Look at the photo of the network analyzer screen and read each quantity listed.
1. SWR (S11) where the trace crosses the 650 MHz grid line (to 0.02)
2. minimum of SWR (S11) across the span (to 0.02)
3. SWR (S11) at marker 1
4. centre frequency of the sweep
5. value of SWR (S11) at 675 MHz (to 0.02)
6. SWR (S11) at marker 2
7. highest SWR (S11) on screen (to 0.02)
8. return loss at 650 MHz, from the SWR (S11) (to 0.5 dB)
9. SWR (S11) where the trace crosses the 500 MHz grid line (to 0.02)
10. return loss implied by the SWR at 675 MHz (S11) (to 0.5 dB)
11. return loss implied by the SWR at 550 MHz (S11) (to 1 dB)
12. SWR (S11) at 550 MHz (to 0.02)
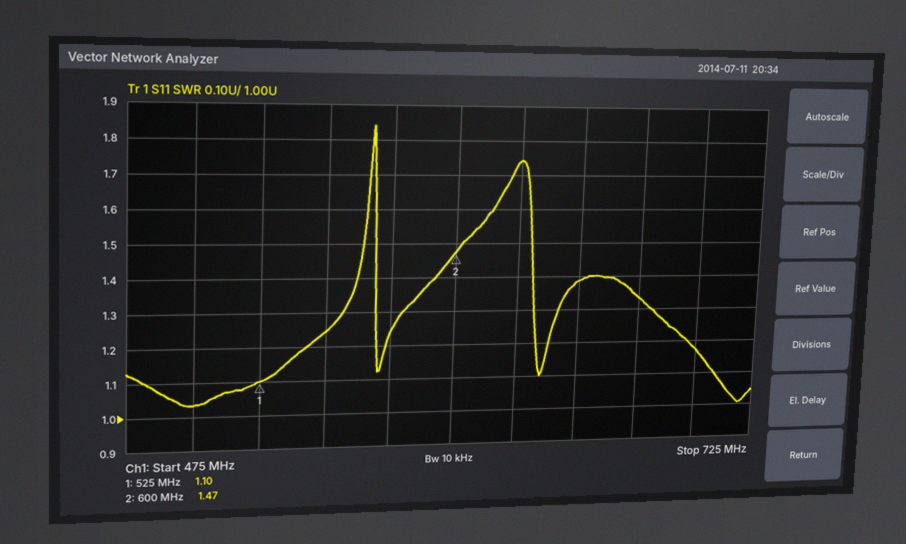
1.38
1.00
1.10
600 MHz
1.34
1.47
1.84
16.0 dB
1.04
17.0 dB
19 dB
1.24
